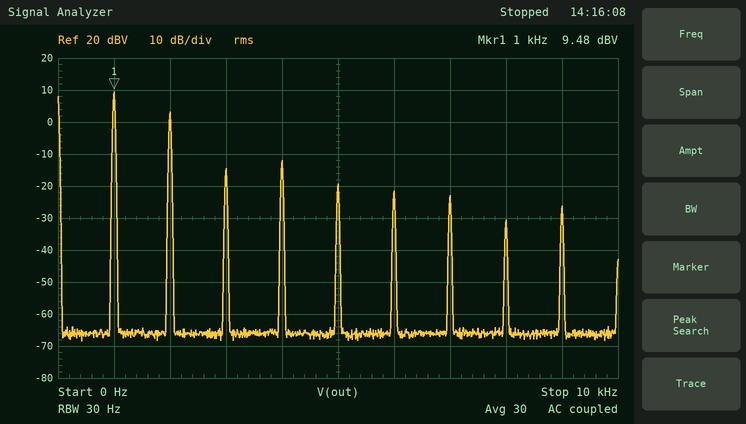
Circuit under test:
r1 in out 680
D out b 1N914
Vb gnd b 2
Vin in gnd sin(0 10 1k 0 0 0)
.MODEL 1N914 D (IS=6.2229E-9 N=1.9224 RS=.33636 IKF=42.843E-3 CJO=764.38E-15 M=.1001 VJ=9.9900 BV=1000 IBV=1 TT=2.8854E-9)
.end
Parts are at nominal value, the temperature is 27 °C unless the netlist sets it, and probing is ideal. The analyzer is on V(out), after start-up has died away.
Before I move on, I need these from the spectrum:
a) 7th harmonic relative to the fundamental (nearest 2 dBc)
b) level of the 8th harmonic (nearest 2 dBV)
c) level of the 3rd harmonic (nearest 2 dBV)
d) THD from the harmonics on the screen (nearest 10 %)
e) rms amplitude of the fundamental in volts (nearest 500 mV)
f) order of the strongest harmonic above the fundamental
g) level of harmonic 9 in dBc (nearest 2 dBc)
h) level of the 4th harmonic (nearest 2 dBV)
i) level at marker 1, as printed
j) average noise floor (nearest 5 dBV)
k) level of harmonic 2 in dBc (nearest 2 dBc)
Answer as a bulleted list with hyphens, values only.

- -32 dBc
- -30 dBV
- -14 dBV
- 50 %
- 3.0 V
- 2
- -36 dBc
- -12 dBV
- 9.48 dBV
- -65 dBV
- -6 dBc
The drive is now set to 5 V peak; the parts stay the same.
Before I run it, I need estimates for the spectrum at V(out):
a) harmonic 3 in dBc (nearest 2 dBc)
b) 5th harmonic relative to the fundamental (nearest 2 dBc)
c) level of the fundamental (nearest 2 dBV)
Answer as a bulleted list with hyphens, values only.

- -16 dBc
- -24 dBc
- 2 dBV
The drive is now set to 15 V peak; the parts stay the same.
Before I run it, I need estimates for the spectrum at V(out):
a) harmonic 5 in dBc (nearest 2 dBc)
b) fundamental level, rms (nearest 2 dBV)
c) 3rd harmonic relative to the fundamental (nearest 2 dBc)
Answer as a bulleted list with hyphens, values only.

- -32 dBc
- 14 dBV
- -28 dBc
